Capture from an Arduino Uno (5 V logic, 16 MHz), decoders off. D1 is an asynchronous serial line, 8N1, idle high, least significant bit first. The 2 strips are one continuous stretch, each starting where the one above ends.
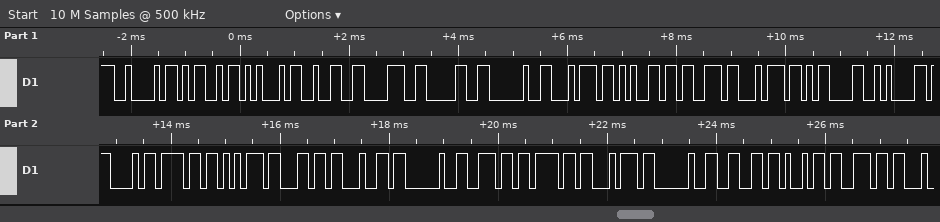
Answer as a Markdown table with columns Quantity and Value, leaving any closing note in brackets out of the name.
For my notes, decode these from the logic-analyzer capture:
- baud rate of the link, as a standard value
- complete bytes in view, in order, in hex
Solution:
| Quantity | Value |
|---|---|
| baud rate of the link, as a standard value | 9600 baud |
| complete bytes in view, in order, in hex | 0x42 0x4D 0x45 0x32 0x38 0x30 0x20 0x74 0x65 0x73 0x74 0x0D 0x0A 0x43 0x6F 0x75 0x6C 0x64 0x20 0x6E 0x6F 0x74 0x20 0x66 0x69 0x6E |
